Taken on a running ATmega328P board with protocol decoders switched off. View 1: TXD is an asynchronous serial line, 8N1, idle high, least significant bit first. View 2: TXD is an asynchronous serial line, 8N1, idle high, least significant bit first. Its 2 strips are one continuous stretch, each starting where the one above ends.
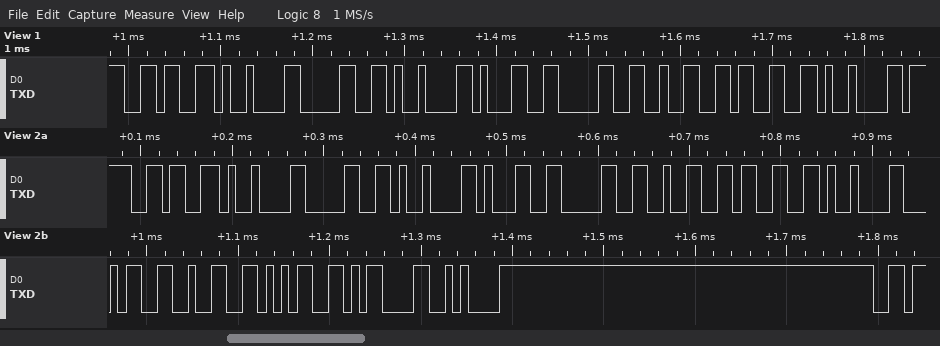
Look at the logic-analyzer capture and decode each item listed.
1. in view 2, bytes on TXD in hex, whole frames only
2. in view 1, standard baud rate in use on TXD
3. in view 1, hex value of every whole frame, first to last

0x36 0x09 0x30 0x09 0x31 0x30 0x32 0x33 0x09 0x34 0x32 0x35 0x0D 0x0A
115200 baud
36 09 30 09 31 30 32 33 09
